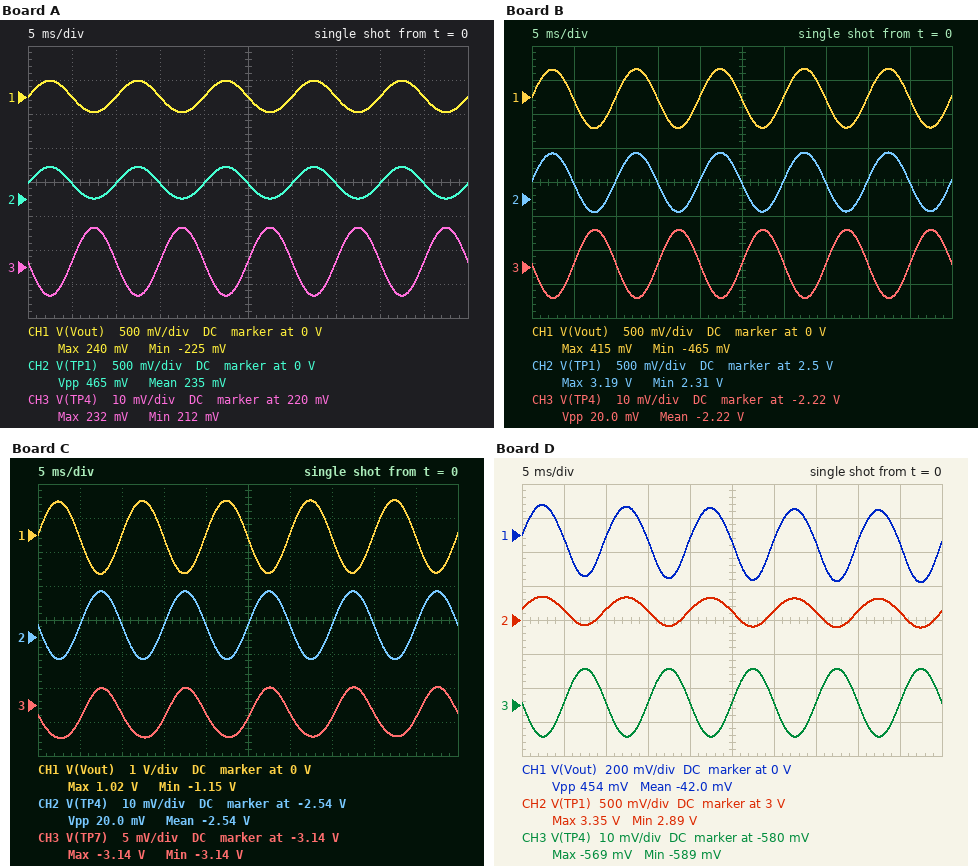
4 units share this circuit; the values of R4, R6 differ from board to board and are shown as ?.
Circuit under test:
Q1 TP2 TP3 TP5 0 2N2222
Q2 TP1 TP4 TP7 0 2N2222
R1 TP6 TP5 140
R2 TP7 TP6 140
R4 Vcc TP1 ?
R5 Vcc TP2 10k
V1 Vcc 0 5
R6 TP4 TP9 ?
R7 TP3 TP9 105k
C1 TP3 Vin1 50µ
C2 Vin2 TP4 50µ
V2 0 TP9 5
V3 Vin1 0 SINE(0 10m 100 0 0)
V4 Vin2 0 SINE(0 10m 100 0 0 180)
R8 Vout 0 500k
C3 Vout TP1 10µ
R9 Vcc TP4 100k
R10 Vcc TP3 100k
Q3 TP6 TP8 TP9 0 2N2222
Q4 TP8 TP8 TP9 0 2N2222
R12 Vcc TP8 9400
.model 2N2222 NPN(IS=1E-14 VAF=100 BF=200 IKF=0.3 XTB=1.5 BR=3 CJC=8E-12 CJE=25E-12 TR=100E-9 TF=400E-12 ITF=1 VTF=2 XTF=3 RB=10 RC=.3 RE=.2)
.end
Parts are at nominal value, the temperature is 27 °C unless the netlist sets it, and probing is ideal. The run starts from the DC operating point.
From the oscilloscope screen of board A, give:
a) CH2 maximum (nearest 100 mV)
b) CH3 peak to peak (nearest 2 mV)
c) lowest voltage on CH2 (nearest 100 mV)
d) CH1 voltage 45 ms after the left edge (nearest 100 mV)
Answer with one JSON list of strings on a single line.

["500 mV", "20 mV", "0 V", "0 V"]
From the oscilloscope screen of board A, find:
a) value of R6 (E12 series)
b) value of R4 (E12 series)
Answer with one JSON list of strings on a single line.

["120 kΩ", "5.6 kΩ"]
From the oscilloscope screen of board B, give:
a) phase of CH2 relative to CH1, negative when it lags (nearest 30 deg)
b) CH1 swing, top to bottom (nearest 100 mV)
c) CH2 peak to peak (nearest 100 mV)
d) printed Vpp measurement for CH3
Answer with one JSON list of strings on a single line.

["0 deg", "900 mV", "900 mV", "20.0 mV"]
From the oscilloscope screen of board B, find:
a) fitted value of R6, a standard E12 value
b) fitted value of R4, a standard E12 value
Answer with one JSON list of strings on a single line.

["39 kΩ", "12 kΩ"]
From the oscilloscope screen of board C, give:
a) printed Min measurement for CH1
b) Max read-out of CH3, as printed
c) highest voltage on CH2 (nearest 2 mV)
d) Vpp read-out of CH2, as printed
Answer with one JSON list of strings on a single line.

["-1.15 V", "-3.14 V", "-2.526 V", "20.0 mV"]
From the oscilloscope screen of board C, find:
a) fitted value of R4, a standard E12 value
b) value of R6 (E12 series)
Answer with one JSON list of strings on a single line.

["33 kΩ", "33 kΩ"]
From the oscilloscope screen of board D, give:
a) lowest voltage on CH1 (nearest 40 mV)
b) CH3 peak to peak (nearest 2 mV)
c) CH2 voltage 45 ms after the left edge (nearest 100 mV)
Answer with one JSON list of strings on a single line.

["-280 mV", "20 mV", "3.1 V"]
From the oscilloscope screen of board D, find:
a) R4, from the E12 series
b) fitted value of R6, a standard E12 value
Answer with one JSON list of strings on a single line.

["4.7 kΩ", "82 kΩ"]
